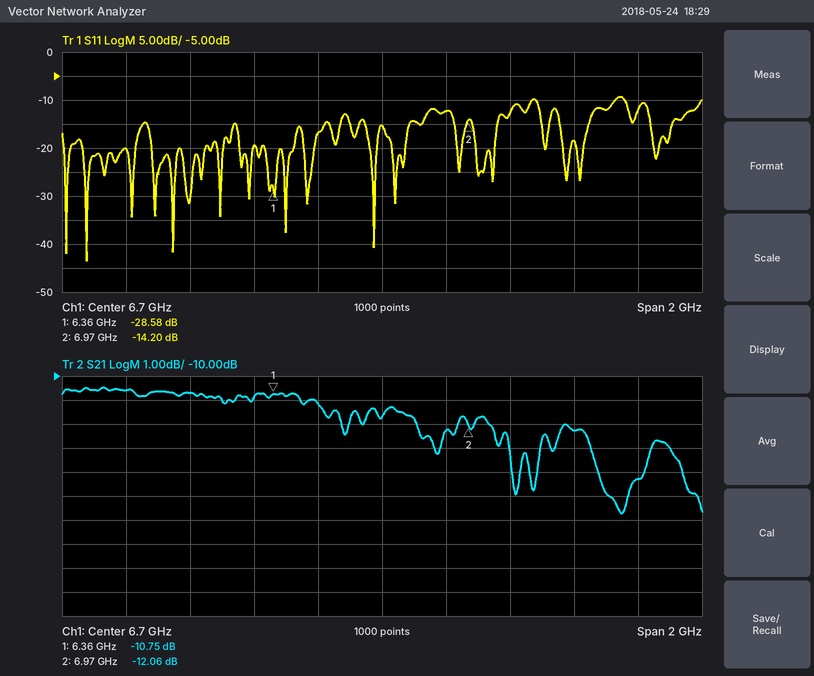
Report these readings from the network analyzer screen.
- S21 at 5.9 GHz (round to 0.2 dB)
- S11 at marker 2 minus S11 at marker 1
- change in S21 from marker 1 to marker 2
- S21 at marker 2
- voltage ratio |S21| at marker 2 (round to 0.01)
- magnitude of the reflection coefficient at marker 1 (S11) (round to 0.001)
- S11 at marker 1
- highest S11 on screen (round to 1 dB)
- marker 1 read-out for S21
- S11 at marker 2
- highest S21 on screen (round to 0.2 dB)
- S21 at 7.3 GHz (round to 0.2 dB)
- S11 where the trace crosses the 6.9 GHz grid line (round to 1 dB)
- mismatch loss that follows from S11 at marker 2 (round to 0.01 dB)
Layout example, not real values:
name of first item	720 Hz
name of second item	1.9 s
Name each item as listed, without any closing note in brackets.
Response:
S21 at 5.9 GHz	-10.6 dB
S11 at marker 2 minus S11 at marker 1	14.38 dB
change in S21 from marker 1 to marker 2	-1.31 dB
S21 at marker 2	-12.06 dB
voltage ratio |S21| at marker 2	0.25
magnitude of the reflection coefficient at marker 1 (S11)	0.037
S11 at marker 1	-28.58 dB
highest S11 on screen	-9 dB
marker 1 read-out for S21	-10.75 dB
S11 at marker 2	-14.20 dB
highest S21 on screen	-10.4 dB
S21 at 7.3 GHz	-12.2 dB
S11 where the trace crosses the 6.9 GHz grid line	-12 dB
mismatch loss that follows from S11 at marker 2	0.17 dB
